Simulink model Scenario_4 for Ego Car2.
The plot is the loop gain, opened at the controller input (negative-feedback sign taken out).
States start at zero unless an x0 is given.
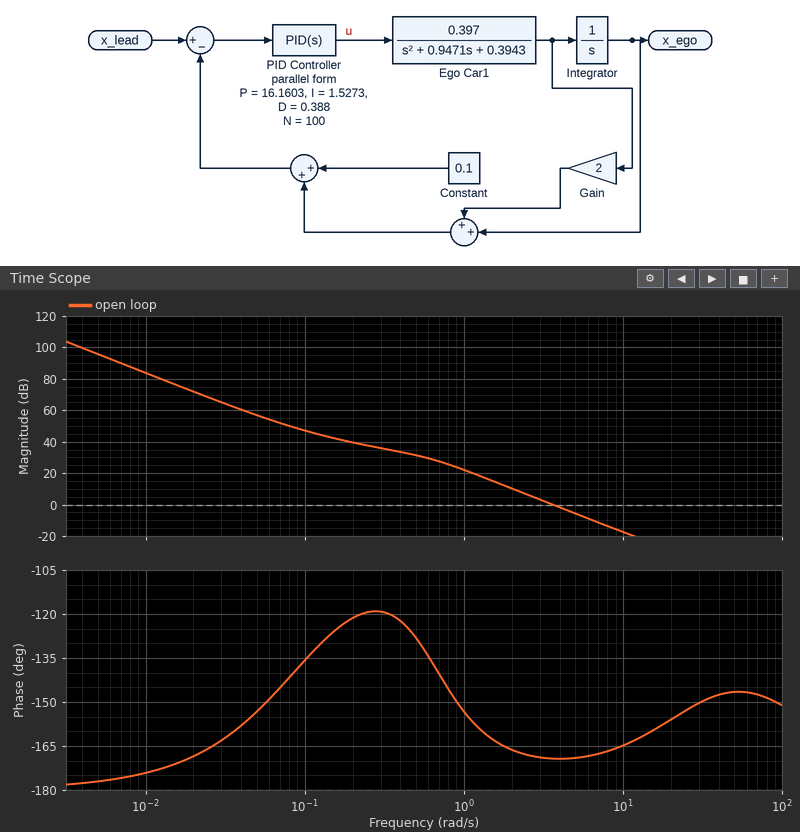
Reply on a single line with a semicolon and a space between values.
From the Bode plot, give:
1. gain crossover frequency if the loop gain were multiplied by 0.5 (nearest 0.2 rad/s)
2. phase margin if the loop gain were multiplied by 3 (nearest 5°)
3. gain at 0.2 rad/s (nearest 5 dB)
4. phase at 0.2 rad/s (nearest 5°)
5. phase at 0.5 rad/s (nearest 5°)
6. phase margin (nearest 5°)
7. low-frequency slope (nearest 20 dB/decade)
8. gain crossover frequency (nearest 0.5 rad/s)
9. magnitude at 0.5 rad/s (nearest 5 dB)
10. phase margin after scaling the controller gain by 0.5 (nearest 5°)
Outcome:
2.6 rad/s; 10°; 40 dB; -120°; -130°; 10°; -40 dB/decade; 3.5 rad/s; 30 dB; 10°
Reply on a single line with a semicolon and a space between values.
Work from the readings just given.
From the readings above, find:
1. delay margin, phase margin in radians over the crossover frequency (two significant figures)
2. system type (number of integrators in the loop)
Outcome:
0.050 s; 2
